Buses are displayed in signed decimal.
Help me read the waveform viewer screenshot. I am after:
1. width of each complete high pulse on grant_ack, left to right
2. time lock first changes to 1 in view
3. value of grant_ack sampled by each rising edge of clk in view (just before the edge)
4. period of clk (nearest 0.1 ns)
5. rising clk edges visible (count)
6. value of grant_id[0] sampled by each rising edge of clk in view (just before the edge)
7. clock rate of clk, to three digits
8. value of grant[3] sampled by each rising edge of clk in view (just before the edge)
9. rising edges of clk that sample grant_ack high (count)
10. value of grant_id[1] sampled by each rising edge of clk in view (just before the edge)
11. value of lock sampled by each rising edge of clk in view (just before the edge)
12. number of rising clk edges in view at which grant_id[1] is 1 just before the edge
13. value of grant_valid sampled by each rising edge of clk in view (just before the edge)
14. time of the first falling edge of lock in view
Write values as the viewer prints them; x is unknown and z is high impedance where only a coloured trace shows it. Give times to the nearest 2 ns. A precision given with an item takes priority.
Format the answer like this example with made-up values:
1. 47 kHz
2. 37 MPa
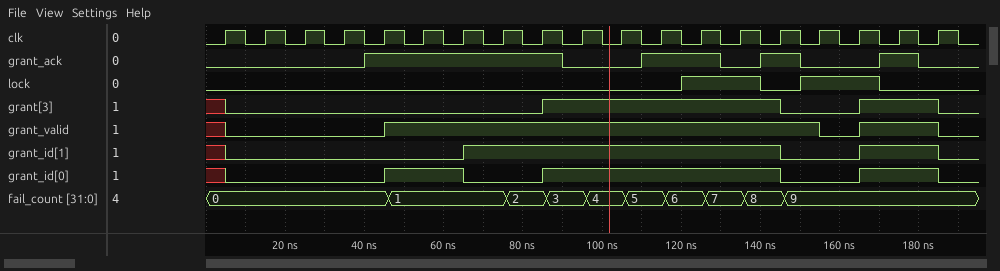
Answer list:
1. 50 ns, 20 ns, 10 ns, 10 ns
2. 120 ns
3. 0 0 0 0 1 1 1 1 1 0 0 1 1 0 1 0 0 1 0
4. 10 ns
5. 19
6. x 0 0 0 0 1 1 0 0 1 1 1 1 1 1 0 0 1 1
7. 100 MHz
8. x 0 0 0 0 0 0 0 0 1 1 1 1 1 1 0 0 1 1
9. 9
10. x 0 0 0 0 0 0 1 1 1 1 1 1 1 1 0 0 1 1
11. 0 0 0 0 0 0 0 0 0 0 0 0 1 1 0 1 1 0 0
12. 10
13. x 0 0 0 0 1 1 1 1 1 1 1 1 1 1 1 0 1 1
14. 140 ns
